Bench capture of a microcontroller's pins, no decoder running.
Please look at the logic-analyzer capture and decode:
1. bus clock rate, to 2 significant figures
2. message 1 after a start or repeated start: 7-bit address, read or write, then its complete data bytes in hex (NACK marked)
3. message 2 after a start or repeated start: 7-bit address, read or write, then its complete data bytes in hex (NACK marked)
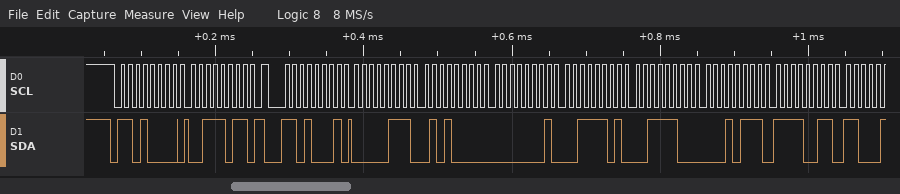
100 kHz
0x68 write: 3B
0x68 read: 07 50 01 3D 3C 17 F3
